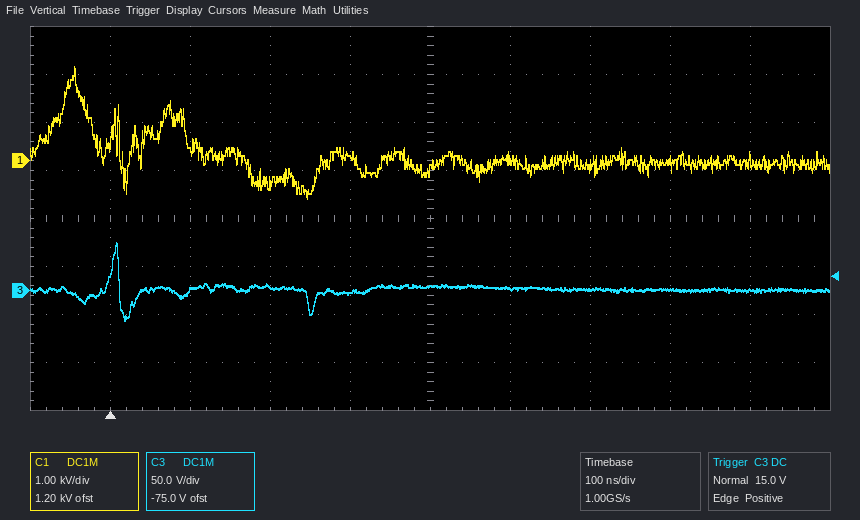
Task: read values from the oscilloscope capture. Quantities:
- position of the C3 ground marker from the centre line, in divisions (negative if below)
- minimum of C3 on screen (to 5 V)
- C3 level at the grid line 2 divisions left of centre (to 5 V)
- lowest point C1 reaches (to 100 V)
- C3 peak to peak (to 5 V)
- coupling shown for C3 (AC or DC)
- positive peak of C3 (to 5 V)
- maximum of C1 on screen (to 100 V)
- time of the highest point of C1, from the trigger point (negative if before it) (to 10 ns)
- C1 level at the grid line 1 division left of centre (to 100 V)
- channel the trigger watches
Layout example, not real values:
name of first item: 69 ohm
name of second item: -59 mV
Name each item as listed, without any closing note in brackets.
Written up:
position of the C3 ground marker from the centre line, in divisions: -1.5 div
minimum of C3 on screen: -30 V
C3 level at the grid line 2 divisions left of centre: 5 V
lowest point C1 reaches: -800 V
C3 peak to peak: 80 V
coupling shown for C3: DC
positive peak of C3: 50 V
maximum of C1 on screen: 2.0 kV
time of the highest point of C1, from the trigger point (negative if before it): -40 ns
C1 level at the grid line 1 division left of centre: 100 V
channel the trigger watches: C3
